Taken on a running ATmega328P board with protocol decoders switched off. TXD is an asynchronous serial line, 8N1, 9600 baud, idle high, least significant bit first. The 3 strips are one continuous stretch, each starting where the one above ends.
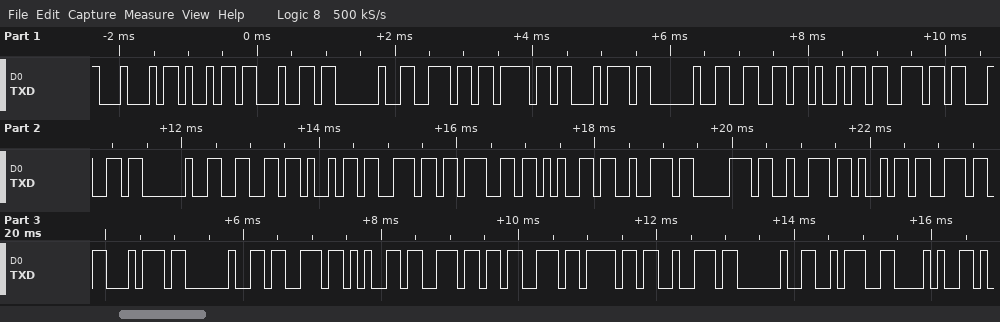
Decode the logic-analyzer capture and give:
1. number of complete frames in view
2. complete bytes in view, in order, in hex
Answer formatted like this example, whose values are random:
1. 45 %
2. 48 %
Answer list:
1. 34
2. 0x44 0x69 0x64 0x20 0x6E 0x6F 0x74 0x20 0x66 0x69 0x6E 0x64 0x20 0x66 0x69 0x6E 0x67 0x65 0x72 0x70 0x72 0x69 0x6E 0x74 0x20 0x73 0x65 0x6E 0x73 0x6F 0x72 0x20 0x3A 0x28
